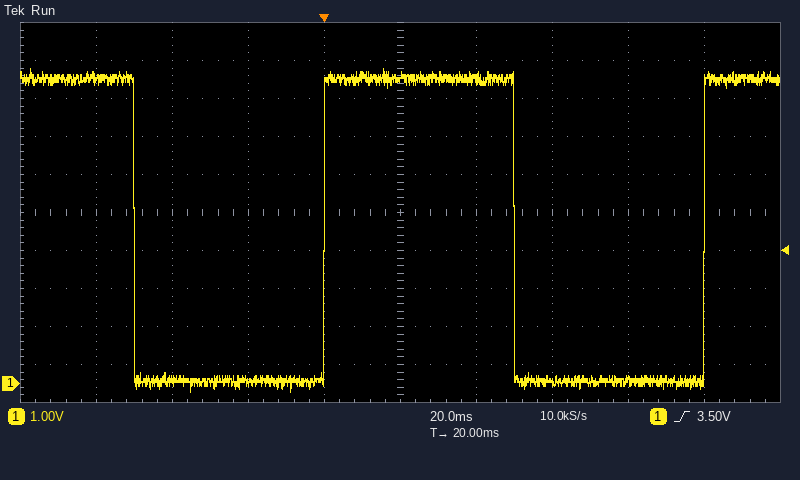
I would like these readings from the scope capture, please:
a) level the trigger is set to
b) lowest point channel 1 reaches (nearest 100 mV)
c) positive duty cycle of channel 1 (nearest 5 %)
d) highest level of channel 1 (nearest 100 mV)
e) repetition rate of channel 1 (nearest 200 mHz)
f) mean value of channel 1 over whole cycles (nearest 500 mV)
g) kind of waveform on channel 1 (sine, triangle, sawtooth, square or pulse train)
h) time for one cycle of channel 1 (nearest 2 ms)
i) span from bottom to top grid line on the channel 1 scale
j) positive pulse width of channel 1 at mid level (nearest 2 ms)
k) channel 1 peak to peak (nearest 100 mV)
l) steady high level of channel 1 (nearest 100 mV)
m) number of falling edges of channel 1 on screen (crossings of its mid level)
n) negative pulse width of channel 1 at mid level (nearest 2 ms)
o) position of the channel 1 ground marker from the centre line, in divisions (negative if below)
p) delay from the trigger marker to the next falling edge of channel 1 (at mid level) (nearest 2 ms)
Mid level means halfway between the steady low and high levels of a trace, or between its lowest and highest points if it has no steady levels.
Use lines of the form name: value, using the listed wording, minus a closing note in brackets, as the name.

level the trigger is set to: 3.50 V
lowest point channel 1 reaches: -200 mV
positive duty cycle of channel 1: 50 %
highest level of channel 1: 8.3 V
repetition rate of channel 1: 10.0 Hz
mean value of channel 1 over whole cycles: 4.0 V
kind of waveform on channel 1: square
time for one cycle of channel 1: 100 ms
span from bottom to top grid line on the channel 1 scale: 10 V
positive pulse width of channel 1 at mid level: 50 ms
channel 1 peak to peak: 8.5 V
steady high level of channel 1: 8.0 V
number of falling edges of channel 1 on screen: 2
negative pulse width of channel 1 at mid level: 50 ms
position of the channel 1 ground marker from the centre line, in divisions: -4.5 div
delay from the trigger marker to the next falling edge of channel 1 (at mid level): 50 ms
